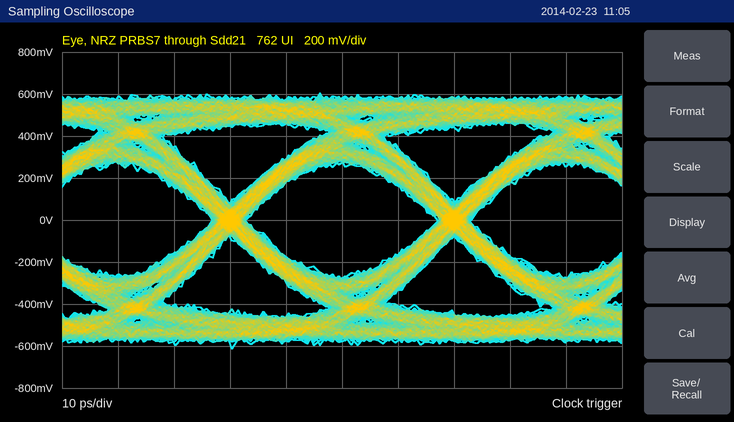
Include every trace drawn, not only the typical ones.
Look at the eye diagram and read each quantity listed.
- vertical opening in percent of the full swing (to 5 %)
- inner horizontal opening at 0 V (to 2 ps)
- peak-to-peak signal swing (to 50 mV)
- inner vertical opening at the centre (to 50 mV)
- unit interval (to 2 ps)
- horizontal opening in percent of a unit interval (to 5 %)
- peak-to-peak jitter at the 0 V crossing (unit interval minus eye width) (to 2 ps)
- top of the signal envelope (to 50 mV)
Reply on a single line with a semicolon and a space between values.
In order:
45 %; 34 ps; 1.20 V; 550 mV; 40 ps; 85 %; 6 ps; 600 mV
